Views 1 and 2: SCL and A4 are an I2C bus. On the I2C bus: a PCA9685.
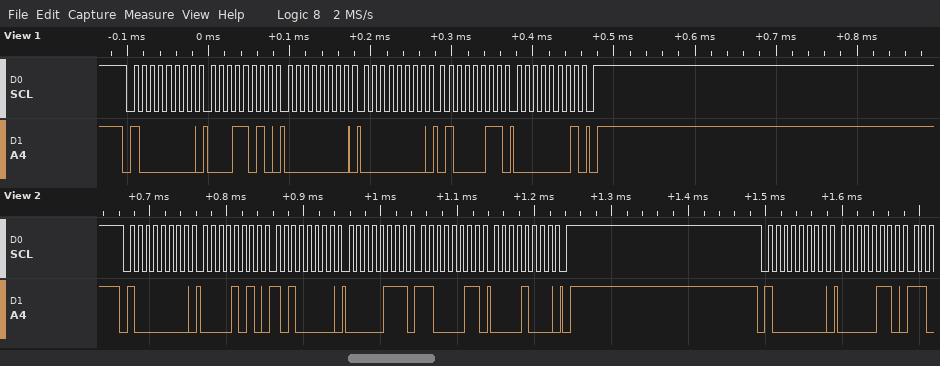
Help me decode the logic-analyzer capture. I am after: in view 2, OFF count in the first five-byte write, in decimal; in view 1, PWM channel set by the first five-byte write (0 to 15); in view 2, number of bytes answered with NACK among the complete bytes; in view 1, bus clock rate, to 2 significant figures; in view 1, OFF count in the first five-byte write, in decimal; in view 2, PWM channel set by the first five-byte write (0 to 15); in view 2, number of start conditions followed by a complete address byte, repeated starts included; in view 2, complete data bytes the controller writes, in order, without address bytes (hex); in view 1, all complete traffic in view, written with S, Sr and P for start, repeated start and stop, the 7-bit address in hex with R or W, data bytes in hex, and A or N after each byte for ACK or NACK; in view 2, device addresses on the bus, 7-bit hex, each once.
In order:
2243
5
0
100 kHz
323
1
2
0A A0 07 C3 08 06
S 40W A 1A A 00 A 00 A 43 A 01 A P
0x40
